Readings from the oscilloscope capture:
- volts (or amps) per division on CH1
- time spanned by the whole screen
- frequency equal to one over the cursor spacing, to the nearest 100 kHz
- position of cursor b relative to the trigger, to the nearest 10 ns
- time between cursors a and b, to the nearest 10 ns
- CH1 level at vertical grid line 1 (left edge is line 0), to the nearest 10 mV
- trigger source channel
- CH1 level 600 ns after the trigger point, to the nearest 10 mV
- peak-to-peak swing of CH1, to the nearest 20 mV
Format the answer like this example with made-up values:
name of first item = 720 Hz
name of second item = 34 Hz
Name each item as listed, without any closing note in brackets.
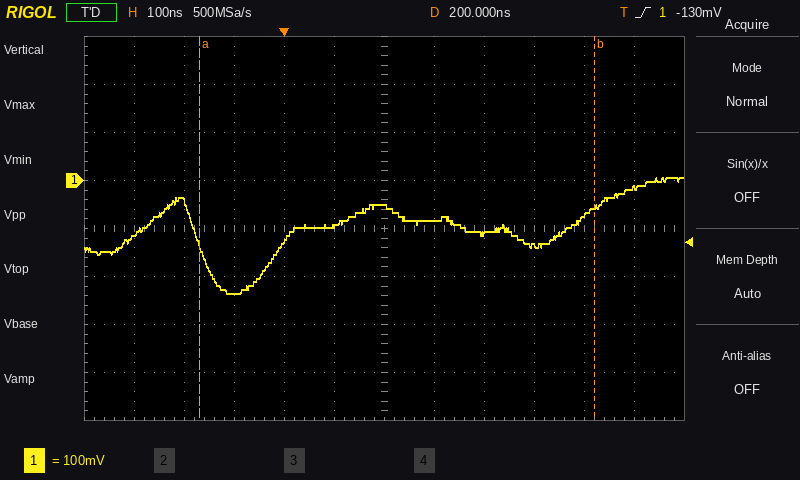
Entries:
volts (or amps) per division on CH1 = 100 mV
time spanned by the whole screen = 1.2 µs
frequency equal to one over the cursor spacing, to the nearest 100 kHz = 1.3 MHz
position of cursor b relative to the trigger, to the nearest 10 ns = +620 ns
time between cursors a and b, to the nearest 10 ns = 790 ns
CH1 level at vertical grid line 1 (left edge is line 0), to the nearest 10 mV = -110 mV
trigger source channel = CH1
CH1 level 600 ns after the trigger point, to the nearest 10 mV = -70 mV
peak-to-peak swing of CH1, to the nearest 20 mV = 240 mV
